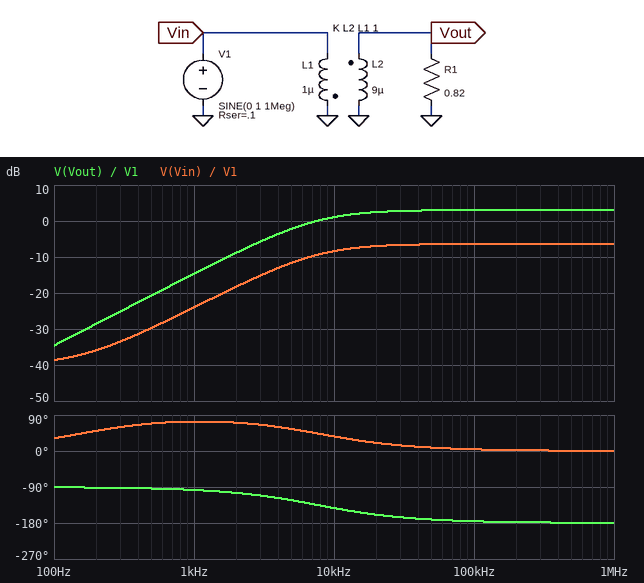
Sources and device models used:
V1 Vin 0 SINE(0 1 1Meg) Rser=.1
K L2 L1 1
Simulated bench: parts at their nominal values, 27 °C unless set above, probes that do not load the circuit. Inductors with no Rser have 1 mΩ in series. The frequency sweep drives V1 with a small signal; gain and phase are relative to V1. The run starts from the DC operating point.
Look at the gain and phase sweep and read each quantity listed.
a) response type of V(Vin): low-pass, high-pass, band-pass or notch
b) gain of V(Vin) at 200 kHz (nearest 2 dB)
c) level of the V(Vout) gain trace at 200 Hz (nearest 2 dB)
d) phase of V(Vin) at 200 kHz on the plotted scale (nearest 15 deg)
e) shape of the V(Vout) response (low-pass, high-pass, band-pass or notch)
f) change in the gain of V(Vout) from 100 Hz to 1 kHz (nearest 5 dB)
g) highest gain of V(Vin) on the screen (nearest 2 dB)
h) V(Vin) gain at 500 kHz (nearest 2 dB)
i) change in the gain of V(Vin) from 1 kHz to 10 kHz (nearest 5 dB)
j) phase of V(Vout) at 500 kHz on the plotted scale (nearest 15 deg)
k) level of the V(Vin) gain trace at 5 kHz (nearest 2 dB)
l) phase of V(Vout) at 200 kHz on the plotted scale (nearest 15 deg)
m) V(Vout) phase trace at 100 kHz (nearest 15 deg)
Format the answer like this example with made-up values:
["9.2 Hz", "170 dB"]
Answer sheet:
["high-pass", "-6 dB", "-28 dB", "0 deg", "high-pass", "20 dB", "-6 dB", "-6 dB", "15 dB", "-180 deg", "-12 dB", "-180 deg", "-180 deg"]
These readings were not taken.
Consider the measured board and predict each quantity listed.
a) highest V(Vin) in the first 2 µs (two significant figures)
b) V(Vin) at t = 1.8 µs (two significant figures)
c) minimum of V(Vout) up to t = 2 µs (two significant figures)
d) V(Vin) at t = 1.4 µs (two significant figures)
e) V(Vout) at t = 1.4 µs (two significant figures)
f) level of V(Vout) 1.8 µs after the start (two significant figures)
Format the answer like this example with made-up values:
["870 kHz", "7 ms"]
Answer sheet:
["480 mV", "-460 mV", "-1.4 V", "280 mV", "-820 mV", "1.4 V"]
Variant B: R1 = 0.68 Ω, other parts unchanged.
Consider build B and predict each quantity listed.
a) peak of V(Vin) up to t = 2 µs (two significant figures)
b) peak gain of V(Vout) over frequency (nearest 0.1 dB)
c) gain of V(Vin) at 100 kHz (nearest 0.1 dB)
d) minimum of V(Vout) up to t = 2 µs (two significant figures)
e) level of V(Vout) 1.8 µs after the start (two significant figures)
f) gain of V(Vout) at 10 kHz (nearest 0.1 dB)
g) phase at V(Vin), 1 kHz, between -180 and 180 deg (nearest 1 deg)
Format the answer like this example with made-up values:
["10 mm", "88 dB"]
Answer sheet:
["430 mV", "2.2 dB", "-7.3 dB", "-1.3 V", "1.2 V", "0.5 dB", "73 deg"]
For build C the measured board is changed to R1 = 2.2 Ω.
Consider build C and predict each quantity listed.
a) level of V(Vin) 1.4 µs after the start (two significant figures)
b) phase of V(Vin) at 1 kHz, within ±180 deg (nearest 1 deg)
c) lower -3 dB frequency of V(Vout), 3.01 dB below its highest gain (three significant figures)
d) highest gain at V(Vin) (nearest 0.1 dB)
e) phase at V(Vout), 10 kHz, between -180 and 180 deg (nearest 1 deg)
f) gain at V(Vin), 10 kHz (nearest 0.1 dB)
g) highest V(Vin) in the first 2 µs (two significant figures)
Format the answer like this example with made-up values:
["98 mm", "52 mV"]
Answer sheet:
["400 mV", "76 deg", "11.4 kHz", "-3.0 dB", "-131 deg", "-6.6 dB", "700 mV"]
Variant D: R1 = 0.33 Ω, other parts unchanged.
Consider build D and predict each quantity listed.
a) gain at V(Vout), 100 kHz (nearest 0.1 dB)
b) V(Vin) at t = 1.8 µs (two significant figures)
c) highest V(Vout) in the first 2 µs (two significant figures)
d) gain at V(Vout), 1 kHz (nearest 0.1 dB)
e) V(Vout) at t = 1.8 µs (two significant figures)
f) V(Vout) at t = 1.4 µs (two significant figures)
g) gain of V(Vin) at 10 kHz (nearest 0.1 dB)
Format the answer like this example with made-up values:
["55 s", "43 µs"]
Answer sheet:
["-2.0 dB", "-260 mV", "800 mV", "-14.8 dB", "760 mV", "-460 mV", "-12.0 dB"]
